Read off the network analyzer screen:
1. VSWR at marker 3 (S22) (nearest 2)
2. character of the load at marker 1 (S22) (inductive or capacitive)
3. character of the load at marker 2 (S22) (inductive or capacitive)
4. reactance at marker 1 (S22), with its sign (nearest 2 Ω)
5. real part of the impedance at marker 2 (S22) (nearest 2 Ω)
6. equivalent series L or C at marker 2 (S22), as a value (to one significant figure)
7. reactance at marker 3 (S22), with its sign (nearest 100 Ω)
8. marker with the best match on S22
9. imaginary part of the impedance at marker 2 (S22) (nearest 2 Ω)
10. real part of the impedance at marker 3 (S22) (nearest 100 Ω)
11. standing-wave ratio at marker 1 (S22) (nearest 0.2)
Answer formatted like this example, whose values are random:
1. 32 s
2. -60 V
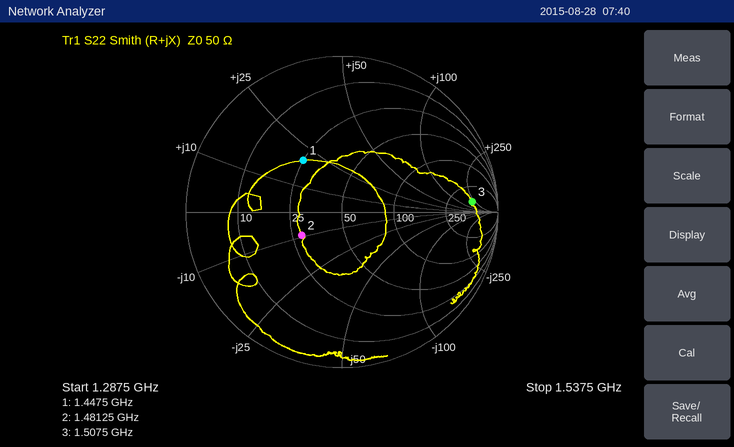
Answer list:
1. 12
2. inductive
3. capacitive
4. +20 Ω
5. 28 Ω
6. 10 pF
7. +200 Ω
8. marker 2
9. -10 Ω
10. 500 Ω
11. 2.4
